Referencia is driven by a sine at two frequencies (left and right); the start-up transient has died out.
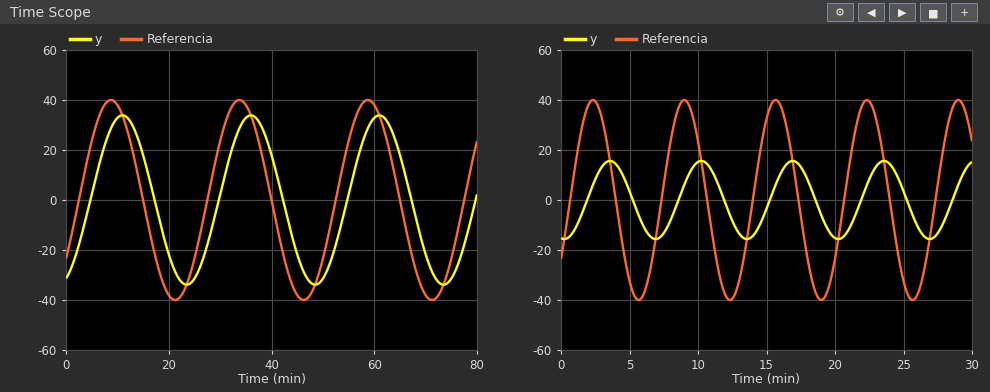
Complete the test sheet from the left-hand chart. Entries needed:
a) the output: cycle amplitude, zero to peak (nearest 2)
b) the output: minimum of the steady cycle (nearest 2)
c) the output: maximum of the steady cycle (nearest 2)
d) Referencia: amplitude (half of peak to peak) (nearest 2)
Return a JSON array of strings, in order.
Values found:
["34", "-34", "34", "40"]
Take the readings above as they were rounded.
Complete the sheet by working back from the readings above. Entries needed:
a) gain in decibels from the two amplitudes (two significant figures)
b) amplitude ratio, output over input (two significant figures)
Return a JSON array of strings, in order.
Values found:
["-1.4 dB", "0.85"]
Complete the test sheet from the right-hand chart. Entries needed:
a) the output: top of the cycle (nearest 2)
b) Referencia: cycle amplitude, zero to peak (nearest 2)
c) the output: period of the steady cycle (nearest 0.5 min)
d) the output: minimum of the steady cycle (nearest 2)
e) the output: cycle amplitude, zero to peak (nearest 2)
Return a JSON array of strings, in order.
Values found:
["16", "40", "6.5 min", "-16", "16"]
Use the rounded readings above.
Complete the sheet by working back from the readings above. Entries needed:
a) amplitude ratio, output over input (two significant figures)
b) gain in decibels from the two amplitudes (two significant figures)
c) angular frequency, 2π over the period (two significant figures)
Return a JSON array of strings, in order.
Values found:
["0.40", "-8.0 dB", "0.97 rad/min"]
